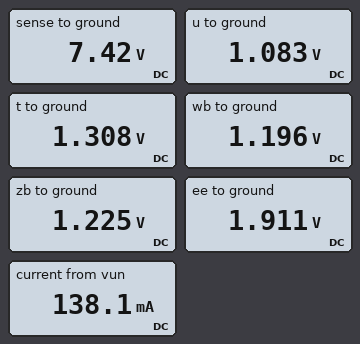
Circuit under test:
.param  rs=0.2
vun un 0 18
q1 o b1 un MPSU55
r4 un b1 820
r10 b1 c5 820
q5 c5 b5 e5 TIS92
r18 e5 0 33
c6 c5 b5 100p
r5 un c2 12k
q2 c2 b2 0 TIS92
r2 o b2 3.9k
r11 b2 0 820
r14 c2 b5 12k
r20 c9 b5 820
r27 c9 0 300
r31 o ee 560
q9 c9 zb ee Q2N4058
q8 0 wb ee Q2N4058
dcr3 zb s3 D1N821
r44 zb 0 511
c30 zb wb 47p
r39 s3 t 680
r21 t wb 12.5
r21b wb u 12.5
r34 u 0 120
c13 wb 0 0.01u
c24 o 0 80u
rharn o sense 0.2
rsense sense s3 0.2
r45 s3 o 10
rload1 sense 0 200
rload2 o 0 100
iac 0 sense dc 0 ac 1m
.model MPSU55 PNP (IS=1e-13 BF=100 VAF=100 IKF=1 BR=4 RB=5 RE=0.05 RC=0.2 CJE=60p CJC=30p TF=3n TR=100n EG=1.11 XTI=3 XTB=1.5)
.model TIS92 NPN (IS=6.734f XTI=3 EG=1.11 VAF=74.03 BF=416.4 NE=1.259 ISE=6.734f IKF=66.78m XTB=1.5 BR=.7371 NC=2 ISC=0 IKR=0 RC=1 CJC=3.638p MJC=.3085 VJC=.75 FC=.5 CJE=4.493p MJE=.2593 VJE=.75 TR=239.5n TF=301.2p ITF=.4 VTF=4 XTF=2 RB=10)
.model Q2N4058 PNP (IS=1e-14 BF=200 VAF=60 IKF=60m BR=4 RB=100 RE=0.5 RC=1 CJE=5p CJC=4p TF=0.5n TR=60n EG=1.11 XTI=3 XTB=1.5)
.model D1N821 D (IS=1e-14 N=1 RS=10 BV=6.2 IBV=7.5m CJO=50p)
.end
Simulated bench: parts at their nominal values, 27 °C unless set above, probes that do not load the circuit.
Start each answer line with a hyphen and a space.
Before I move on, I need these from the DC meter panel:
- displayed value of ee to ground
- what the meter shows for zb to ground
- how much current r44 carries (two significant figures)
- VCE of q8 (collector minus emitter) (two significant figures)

- 1.911 V
- 1.225 V
- 2.4 mA
- -1.9 V
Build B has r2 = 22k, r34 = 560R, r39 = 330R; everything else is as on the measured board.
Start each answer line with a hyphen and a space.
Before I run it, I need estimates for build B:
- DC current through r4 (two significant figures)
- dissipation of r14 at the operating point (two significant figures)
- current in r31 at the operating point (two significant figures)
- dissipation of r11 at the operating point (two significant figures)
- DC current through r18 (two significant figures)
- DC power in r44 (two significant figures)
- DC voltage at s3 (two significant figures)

- 960 µA
- 4.2 mW
- 10 mA
- 480 µW
- 5.1 mA
- 240 mW
- 17 V
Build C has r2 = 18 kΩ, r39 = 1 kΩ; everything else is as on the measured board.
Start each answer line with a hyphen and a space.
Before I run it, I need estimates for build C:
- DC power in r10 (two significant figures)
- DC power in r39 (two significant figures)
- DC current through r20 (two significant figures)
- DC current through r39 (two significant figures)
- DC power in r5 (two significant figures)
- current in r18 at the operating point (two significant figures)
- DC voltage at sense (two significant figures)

- 6.8 mW
- 75 mW
- 700 µA
- 8.7 mA
- 6.2 mW
- 2.9 mA
- 10 V
